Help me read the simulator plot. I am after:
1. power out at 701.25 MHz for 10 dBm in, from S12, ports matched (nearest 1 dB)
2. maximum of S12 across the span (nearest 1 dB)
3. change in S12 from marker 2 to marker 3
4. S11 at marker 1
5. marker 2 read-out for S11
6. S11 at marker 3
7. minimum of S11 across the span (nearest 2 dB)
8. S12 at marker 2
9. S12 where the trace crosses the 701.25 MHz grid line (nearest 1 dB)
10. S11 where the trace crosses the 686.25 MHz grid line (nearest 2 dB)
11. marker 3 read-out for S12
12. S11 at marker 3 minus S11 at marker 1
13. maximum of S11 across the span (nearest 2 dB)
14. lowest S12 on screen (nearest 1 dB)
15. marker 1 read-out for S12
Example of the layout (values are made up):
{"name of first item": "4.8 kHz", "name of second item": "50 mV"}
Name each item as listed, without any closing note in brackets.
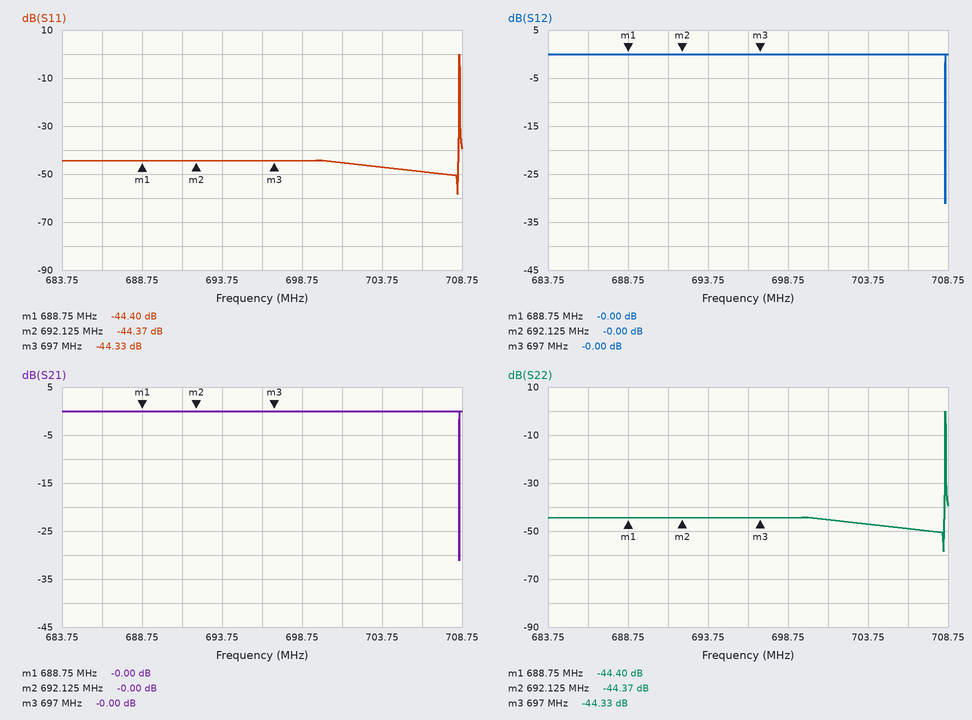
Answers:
{"power out at 701.25 MHz for 10 dBm in, from S12, ports matched": "10 dBm", "maximum of S12 across the span": "0 dB", "change in S12 from marker 2 to marker 3": "0.00 dB", "S11 at marker 1": "-44.40 dB", "marker 2 read-out for S11": "-44.37 dB", "S11 at marker 3": "-44.33 dB", "minimum of S11 across the span": "-58 dB", "S12 at marker 2": "-0.00 dB", "S12 where the trace crosses the 701.25 MHz grid line": "0 dB", "S11 where the trace crosses the 686.25 MHz grid line": "-44 dB", "marker 3 read-out for S12": "-0.00 dB", "S11 at marker 3 minus S11 at marker 1": "0.07 dB", "maximum of S11 across the span": "0 dB", "lowest S12 on screen": "-31 dB", "marker 1 read-out for S12": "-0.00 dB"}
